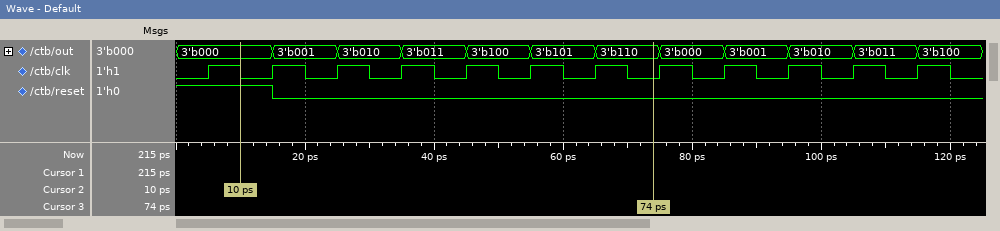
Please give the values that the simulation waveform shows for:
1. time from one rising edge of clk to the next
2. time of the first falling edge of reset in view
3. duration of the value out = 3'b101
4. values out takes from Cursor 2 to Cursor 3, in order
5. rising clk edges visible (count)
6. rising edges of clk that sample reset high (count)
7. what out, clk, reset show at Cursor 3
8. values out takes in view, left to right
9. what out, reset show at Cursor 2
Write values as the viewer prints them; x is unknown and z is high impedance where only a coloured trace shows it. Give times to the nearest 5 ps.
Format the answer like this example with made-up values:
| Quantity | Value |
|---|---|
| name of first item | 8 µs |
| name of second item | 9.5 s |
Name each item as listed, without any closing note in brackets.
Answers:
| Quantity | Value |
|---|---|
| time from one rising edge of clk to the next | 10 ps |
| time of the first falling edge of reset in view | 15 ps |
| duration of the value out = 3'b101 | 10 ps |
| values out takes from Cursor 2 to Cursor 3, in order | 3'b000, 3'b001, 3'b010, 3'b011, 3'b100, 3'b101, 3'b110 |
| rising clk edges visible | 12 |
| rising edges of clk that sample reset high | 2 |
| what out, clk, reset show at Cursor 3 | out=3'b110, clk=0, reset=0 |
| values out takes in view, left to right | 3'b000, 3'b001, 3'b010, 3'b011, 3'b100, 3'b101, 3'b110, 3'b000, 3'b001, 3'b010, 3'b011, 3'b100 |
| what out, reset show at Cursor 2 | out=3'b000, reset=1 |
